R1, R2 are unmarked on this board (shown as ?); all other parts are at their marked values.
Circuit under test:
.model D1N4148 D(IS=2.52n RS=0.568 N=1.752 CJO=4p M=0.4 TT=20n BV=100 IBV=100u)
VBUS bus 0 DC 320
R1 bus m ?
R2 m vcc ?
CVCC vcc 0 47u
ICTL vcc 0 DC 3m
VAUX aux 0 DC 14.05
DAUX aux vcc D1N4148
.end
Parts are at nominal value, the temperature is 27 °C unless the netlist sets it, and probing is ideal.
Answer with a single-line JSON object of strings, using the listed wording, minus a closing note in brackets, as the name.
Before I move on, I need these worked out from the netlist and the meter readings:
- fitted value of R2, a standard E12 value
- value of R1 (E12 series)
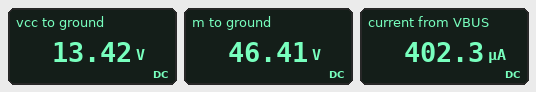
{"fitted value of R2, a standard E12 value": "82 kΩ", "value of R1": "680 kΩ"}
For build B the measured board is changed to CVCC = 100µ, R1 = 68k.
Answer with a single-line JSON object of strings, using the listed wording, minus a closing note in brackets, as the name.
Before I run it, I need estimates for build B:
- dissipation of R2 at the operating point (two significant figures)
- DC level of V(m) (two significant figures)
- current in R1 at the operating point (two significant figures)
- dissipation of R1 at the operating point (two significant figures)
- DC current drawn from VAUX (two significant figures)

{"dissipation of R2 at the operating point": "340 mW", "DC level of V(m)": "180 V", "current in R1 at the operating point": "2.0 mA", "dissipation of R1 at the operating point": "280 mW", "DC current drawn from VAUX": "960 µA"}
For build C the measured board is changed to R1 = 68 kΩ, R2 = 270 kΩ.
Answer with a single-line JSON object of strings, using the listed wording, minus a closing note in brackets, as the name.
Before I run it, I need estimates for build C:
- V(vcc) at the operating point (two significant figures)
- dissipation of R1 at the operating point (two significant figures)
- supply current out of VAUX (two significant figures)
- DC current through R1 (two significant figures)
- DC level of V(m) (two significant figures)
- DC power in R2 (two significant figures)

{"V(vcc) at the operating point": "13 V", "dissipation of R1 at the operating point": "56 mW", "supply current out of VAUX": "2.1 mA", "DC current through R1": "910 µA", "DC level of V(m)": "260 V", "DC power in R2": "220 mW"}
